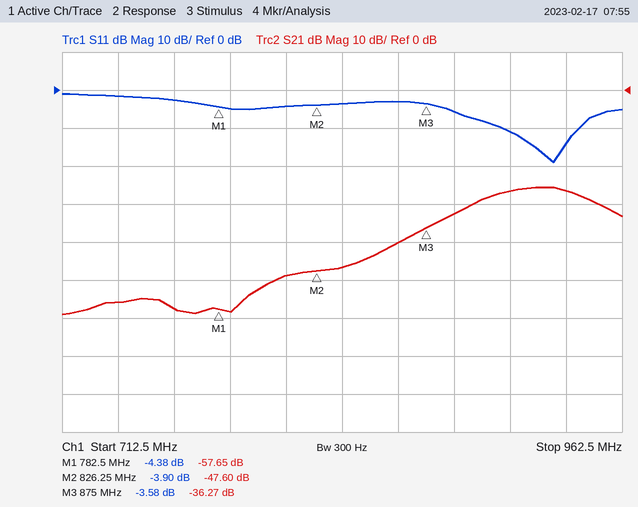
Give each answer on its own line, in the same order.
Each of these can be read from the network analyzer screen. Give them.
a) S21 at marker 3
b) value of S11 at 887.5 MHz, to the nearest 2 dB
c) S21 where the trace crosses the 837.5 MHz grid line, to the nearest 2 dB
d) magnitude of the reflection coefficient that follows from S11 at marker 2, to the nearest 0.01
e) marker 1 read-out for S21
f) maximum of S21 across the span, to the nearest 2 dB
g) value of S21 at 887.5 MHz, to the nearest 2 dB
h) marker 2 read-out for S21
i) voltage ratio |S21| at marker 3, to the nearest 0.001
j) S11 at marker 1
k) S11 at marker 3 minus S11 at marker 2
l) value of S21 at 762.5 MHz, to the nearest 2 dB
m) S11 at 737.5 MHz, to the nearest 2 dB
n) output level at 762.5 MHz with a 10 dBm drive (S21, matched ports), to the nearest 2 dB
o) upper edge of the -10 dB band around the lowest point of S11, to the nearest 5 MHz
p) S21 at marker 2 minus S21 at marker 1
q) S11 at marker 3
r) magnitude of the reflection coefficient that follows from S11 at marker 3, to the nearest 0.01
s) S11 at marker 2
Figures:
-36.27 dB
-6 dB
-46 dB
0.64
-57.65 dB
-26 dB
-32 dB
-47.60 dB
0.015
-4.38 dB
0.32 dB
-58 dB
-2 dB
-48 dBm
945 MHz
10.05 dB
-3.58 dB
0.66
-3.90 dB
